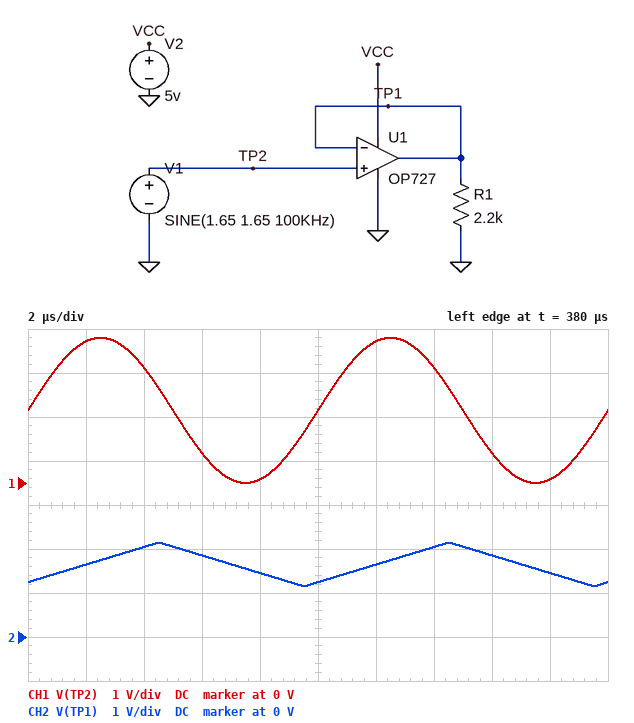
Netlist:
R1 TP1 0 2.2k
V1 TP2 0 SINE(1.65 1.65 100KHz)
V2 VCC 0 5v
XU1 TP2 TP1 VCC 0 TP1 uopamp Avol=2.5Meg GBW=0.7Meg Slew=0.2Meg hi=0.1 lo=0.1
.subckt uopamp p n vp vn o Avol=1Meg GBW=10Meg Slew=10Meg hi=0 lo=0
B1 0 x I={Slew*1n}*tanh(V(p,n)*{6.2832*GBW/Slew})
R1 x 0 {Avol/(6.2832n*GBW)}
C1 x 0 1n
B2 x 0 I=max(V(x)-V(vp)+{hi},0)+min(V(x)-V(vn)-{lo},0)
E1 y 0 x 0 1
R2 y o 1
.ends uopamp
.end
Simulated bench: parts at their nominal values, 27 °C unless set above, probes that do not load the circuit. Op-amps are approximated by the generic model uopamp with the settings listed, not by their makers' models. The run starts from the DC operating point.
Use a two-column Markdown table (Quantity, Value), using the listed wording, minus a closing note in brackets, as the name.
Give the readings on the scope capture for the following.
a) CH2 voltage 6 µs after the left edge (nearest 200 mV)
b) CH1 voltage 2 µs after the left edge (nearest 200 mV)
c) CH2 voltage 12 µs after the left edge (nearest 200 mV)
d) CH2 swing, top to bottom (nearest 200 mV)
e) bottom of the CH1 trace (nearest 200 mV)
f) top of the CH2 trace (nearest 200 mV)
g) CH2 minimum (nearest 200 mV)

| Quantity | Value |
|---|---|
| CH2 voltage 6 µs after the left edge | 1.8 V |
| CH1 voltage 2 µs after the left edge | 3.2 V |
| CH2 voltage 12 µs after the left edge | 1.6 V |
| CH2 swing, top to bottom | 1.0 V |
| bottom of the CH1 trace | 0 V |
| top of the CH2 trace | 2.2 V |
| CH2 minimum | 1.2 V |
